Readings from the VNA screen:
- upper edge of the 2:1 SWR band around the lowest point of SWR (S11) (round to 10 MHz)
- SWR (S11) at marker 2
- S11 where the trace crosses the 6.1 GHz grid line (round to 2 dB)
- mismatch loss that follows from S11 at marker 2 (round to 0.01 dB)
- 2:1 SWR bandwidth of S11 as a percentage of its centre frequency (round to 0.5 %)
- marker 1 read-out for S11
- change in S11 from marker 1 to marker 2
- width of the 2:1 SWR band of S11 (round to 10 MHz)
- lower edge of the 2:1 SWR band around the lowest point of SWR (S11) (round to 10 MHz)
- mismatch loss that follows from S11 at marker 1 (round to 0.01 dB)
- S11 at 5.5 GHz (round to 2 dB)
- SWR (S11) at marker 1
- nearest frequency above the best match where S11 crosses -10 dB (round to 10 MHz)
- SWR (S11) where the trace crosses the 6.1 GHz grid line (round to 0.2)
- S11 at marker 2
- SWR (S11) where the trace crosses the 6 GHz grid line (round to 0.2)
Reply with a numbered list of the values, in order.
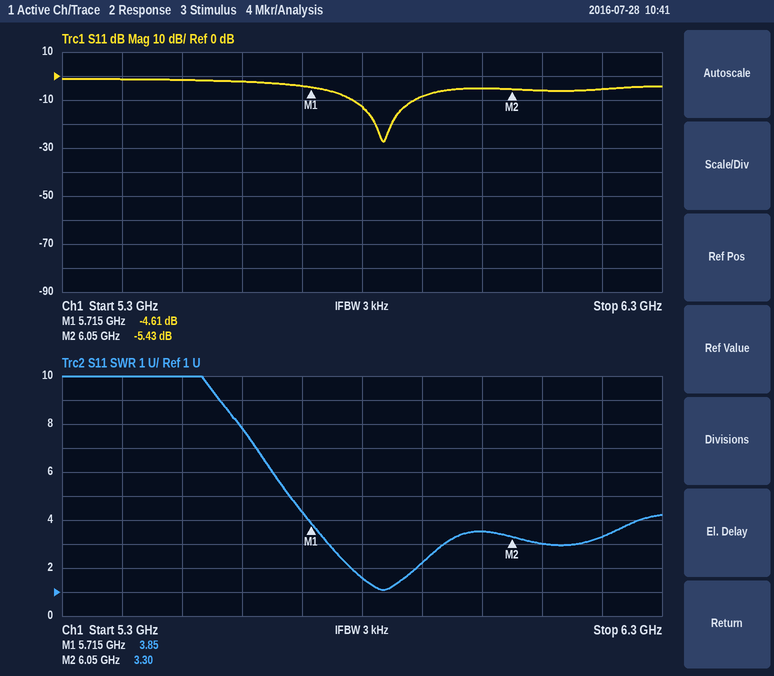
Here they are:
1. 5.89 GHz
2. 3.30
3. -6 dB
4. 1.47 dB
5. 2.0 %
6. -4.61 dB
7. -0.82 dB
8. 110 MHz
9. 5.78 GHz
10. 1.84 dB
11. -2 dB
12. 3.85
13. 5.89 GHz
14. 3.0
15. -5.43 dB
16. 3.6
